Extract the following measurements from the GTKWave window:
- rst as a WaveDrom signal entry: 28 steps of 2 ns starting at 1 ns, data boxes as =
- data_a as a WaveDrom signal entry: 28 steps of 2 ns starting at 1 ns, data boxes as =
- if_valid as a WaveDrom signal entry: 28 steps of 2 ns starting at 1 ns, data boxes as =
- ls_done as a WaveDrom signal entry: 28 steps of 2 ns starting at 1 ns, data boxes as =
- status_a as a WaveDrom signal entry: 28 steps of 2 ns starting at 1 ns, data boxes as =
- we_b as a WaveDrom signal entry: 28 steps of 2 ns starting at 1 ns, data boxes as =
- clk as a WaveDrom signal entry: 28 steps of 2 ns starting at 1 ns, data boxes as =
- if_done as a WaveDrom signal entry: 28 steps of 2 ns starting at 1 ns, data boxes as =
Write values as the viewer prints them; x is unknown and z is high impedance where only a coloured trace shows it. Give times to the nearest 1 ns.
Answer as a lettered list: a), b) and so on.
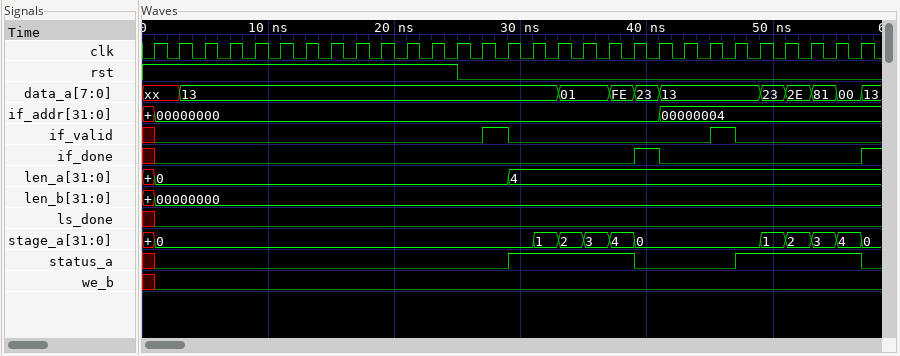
a) {name: 'rst', wave: '1...........0...............'}
b) {name: 'data_a', wave: 'x=..............=.===...====', data: '13 01 FE 23 13 23 2E 81 00'}
c) {name: 'if_valid', wave: '0............10.......10....'}
d) {name: 'ls_done', wave: '0...........................'}
e) {name: 'status_a', wave: '0.............1....0...1....'}
f) {name: 'we_b', wave: '0...........................'}
g) {name: 'clk', wave: 'p...........................'}
h) {name: 'if_done', wave: '0..................10.......'}
